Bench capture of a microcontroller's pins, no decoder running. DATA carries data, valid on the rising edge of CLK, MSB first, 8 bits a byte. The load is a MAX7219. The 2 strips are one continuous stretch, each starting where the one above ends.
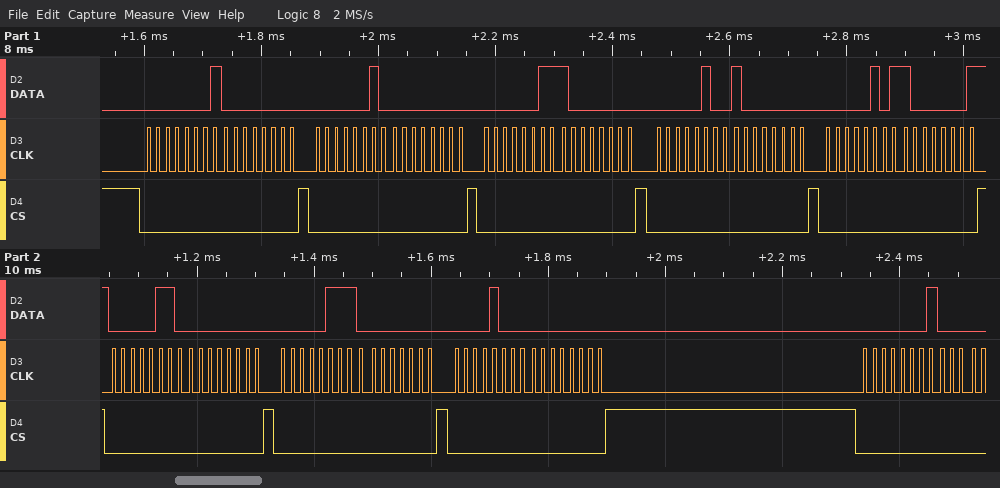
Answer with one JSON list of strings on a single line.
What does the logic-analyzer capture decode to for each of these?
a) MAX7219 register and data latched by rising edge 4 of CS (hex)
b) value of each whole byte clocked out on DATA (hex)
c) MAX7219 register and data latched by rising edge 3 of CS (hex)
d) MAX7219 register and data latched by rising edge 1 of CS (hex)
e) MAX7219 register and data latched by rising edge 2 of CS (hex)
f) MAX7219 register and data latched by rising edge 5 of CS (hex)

["register 0x4, data 0x80", "0x01 0x00 0x02 0x00 0x03 0x80 0x04 0x80 0x05 0x81 0x06 0x00 0x07 0x00 0x08 0x00 0x01", "register 0x3, data 0x80", "register 0x1, data 0x00", "register 0x2, data 0x00", "register 0x5, data 0x81"]
